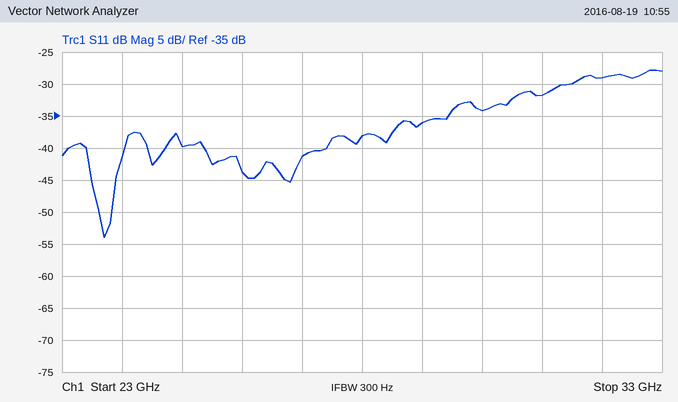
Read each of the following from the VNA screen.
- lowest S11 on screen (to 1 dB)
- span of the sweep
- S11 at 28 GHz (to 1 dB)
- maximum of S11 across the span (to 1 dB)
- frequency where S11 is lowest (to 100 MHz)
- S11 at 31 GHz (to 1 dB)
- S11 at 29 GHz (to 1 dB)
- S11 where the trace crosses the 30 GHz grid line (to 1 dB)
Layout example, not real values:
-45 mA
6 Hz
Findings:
-54 dB
10 GHz
-38 dB
-28 dB
23.7 GHz
-32 dB
-36 dB
-34 dB
